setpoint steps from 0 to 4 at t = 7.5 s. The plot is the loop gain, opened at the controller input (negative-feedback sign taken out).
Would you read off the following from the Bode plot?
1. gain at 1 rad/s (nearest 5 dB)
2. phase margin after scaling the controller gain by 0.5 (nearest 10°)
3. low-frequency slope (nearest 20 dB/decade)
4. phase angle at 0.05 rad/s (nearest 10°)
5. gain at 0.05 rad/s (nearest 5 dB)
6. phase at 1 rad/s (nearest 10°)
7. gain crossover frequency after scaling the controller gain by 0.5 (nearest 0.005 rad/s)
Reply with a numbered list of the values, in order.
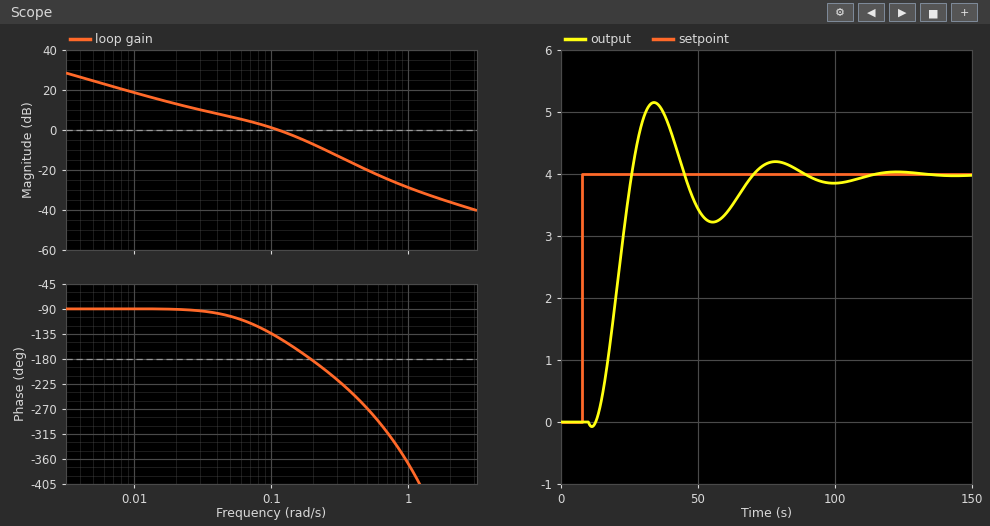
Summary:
1. -30 dB
2. 70°
3. -20 dB/decade
4. -100°
5. 5 dB
6. -370°
7. 0.055 rad/s
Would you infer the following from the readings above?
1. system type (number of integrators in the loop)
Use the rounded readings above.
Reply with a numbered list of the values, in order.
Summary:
1. 1
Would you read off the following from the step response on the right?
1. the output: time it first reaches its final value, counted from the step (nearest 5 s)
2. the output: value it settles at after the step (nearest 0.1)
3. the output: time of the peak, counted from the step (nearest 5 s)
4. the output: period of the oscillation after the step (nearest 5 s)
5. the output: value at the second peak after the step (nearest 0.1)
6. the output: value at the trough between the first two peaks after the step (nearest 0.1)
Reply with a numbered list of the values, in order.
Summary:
1. 20 s
2. 4.0
3. 25 s
4. 45 s
5. 4.2
6. 3.2
